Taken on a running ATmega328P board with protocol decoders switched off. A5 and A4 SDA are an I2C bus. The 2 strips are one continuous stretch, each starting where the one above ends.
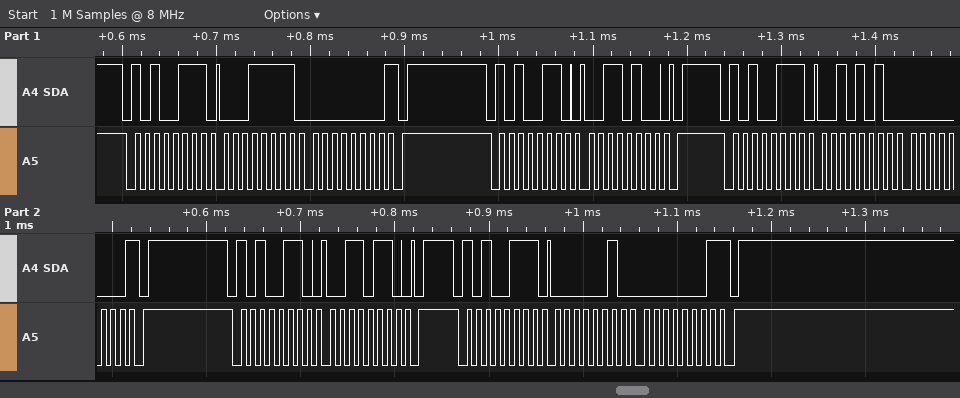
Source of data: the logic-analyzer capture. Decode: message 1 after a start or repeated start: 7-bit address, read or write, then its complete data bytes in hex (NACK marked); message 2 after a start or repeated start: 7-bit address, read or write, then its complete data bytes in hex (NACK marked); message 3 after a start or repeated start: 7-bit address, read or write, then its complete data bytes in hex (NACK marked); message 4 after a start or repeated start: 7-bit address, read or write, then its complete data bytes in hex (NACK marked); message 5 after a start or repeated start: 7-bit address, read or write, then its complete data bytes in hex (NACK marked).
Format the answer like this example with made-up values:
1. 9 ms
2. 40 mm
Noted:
1. 0x53 read: 1F 00 NACK
2. 0x53 write: 34
3. 0x53 read: 2A 00 NACK
4. 0x53 write: 36
5. 0x53 read: 02 01 NACK
